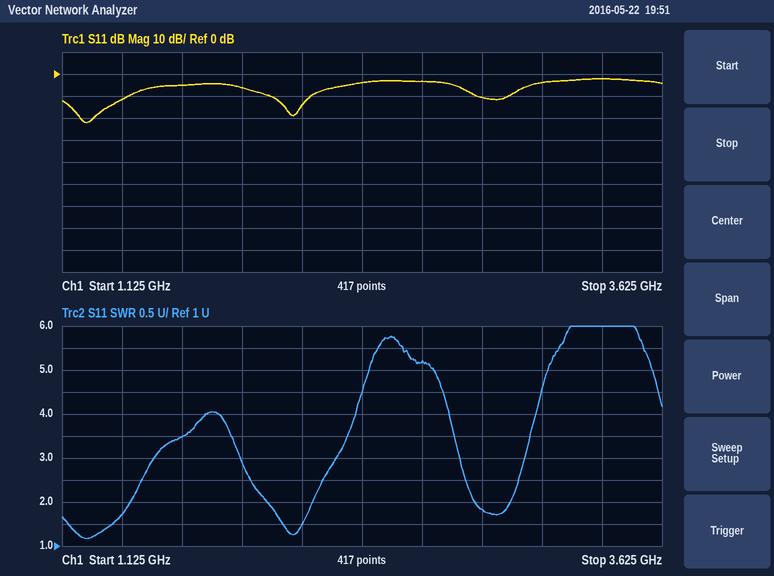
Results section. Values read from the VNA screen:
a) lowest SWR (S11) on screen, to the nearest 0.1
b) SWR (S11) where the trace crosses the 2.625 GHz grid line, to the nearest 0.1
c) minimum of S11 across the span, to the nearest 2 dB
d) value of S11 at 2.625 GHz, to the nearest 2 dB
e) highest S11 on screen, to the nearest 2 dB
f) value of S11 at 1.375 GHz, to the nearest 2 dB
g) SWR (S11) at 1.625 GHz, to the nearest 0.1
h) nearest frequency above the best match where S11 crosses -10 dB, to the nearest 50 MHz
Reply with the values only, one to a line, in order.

1.2
5.2
-22 dB
-4 dB
-2 dB
-12 dB
3.5
1.40 GHz
